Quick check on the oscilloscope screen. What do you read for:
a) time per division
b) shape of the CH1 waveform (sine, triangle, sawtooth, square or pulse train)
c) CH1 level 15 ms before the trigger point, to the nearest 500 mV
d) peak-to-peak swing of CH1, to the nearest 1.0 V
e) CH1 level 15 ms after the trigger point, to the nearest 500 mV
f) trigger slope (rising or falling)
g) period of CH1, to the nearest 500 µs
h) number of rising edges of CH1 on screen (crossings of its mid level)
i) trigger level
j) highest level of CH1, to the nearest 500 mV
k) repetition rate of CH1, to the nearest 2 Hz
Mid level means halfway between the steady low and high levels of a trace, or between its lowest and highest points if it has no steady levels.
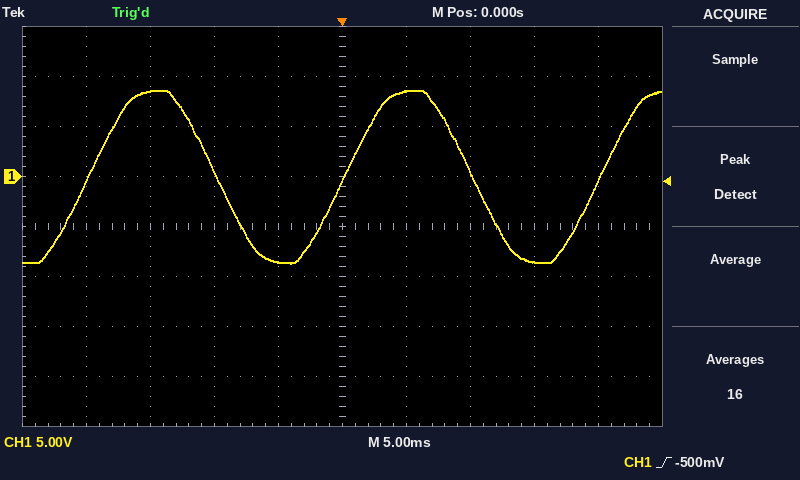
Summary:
5 ms
sine
8.5 V
17.0 V
-8.5 V
rising
20.0 ms
3
-500 mV
8.5 V
50 Hz
